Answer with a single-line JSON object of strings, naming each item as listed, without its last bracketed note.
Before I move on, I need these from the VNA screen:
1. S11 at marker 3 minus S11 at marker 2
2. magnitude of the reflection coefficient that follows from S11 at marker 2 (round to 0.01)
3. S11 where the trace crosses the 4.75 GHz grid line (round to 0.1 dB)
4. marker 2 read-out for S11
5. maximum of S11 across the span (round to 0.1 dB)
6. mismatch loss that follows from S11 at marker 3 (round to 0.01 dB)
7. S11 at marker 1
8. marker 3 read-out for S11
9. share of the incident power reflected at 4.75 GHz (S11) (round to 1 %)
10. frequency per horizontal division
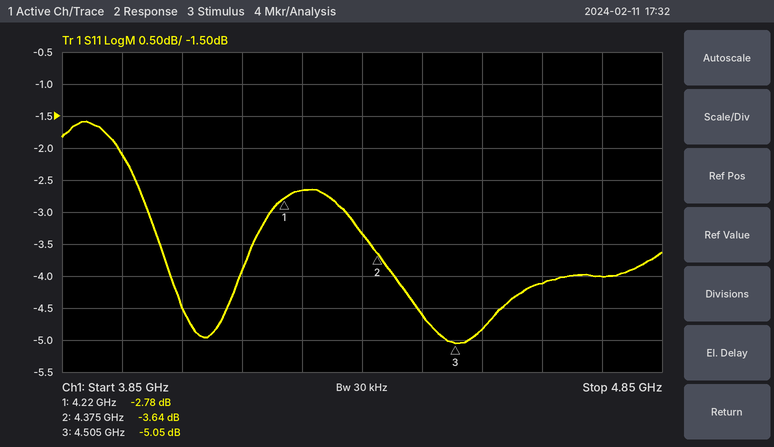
{"S11 at marker 3 minus S11 at marker 2": "-1.41 dB", "magnitude of the reflection coefficient that follows from S11 at marker 2": "0.66", "S11 where the trace crosses the 4.75 GHz grid line": "-4.0 dB", "marker 2 read-out for S11": "-3.64 dB", "maximum of S11 across the span": "-1.6 dB", "mismatch loss that follows from S11 at marker 3": "1.63 dB", "S11 at marker 1": "-2.78 dB", "marker 3 read-out for S11": "-5.05 dB", "share of the incident power reflected at 4.75 GHz (S11)": "40 %", "frequency per horizontal division": "100 MHz"}
